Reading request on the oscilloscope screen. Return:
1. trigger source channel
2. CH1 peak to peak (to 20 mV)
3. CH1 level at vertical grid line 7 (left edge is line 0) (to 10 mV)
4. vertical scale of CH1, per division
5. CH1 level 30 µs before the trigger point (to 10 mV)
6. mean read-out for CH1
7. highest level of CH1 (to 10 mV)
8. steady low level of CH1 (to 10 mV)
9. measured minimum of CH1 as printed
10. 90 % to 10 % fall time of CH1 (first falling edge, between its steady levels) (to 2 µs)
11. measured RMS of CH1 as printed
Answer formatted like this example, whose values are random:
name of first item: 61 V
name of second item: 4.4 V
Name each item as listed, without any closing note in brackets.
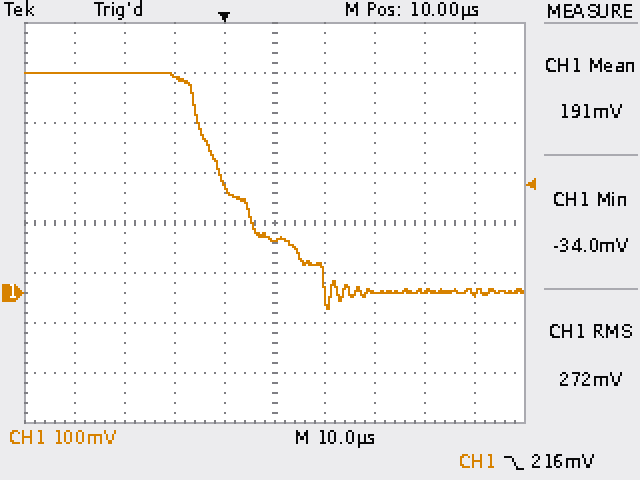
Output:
trigger source channel: CH1
CH1 peak to peak: 480 mV
CH1 level at vertical grid line 7 (left edge is line 0): 0 mV
vertical scale of CH1, per division: 100 mV
CH1 level 30 µs before the trigger point: 440 mV
mean read-out for CH1: 191 mV
highest level of CH1: 440 mV
steady low level of CH1: 0 mV
measured minimum of CH1 as printed: -34.0 mV
90 % to 10 % fall time of CH1 (first falling edge, between its steady levels): 26 µs
measured RMS of CH1 as printed: 272 mV
